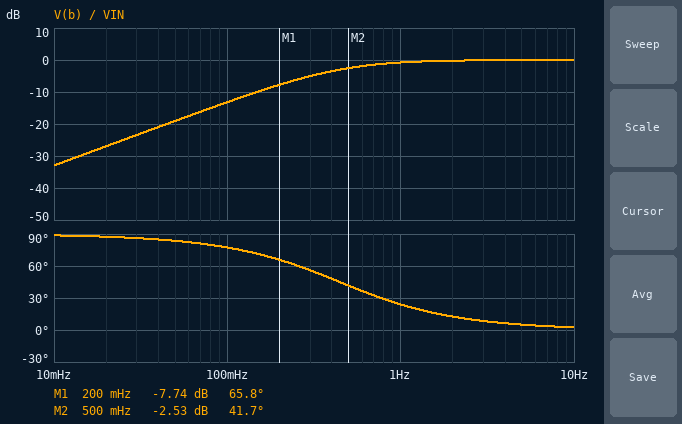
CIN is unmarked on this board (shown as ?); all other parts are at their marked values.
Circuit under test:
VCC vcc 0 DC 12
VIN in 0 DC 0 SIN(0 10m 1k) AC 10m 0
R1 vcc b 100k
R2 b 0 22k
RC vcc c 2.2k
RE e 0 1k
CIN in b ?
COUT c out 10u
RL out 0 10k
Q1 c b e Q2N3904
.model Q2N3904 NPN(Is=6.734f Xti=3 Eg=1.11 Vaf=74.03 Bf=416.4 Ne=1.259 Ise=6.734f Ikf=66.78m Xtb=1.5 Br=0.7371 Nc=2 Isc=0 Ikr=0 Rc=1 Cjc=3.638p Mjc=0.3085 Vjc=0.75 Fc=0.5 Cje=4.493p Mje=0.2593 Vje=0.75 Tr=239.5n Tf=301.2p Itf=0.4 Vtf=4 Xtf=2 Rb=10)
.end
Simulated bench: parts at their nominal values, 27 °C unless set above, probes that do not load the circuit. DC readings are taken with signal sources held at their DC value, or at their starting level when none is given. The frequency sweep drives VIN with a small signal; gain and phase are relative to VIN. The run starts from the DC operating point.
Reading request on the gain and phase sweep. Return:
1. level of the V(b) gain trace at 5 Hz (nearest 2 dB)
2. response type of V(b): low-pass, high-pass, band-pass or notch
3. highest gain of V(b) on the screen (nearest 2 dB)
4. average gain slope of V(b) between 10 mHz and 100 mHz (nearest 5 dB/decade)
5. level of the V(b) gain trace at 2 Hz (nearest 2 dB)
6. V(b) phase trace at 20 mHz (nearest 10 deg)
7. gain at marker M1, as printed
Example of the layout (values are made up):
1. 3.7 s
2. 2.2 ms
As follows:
1. 0 dB
2. high-pass
3. 0 dB
4. 20 dB/decade
5. 0 dB
6. 90 deg
7. -7.74 dB
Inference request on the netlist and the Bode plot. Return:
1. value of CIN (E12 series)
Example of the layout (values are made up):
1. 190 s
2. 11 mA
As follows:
1. 22 µF
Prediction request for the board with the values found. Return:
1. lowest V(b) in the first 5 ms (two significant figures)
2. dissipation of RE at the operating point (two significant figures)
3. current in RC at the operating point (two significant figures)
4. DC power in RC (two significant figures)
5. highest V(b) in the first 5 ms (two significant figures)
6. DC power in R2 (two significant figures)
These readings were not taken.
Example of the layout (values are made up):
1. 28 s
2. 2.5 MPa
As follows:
1. 2.0 V
2. 1.8 mW
3. 1.3 mA
4. 3.9 mW
5. 2.0 V
6. 180 µW
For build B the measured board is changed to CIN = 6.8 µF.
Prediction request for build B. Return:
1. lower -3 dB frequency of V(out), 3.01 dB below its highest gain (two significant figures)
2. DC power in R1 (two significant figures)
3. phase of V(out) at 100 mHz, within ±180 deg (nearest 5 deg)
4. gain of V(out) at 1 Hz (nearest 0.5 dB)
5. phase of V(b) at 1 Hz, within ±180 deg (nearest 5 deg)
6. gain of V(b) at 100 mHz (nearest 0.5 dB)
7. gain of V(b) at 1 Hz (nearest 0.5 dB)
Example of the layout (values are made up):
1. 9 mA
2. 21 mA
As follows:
1. 2.1 Hz
2. 1.0 mW
3. -10 deg
4. -4.5 dB
5. 55 deg
6. -23.0 dB
7. -5.0 dB
